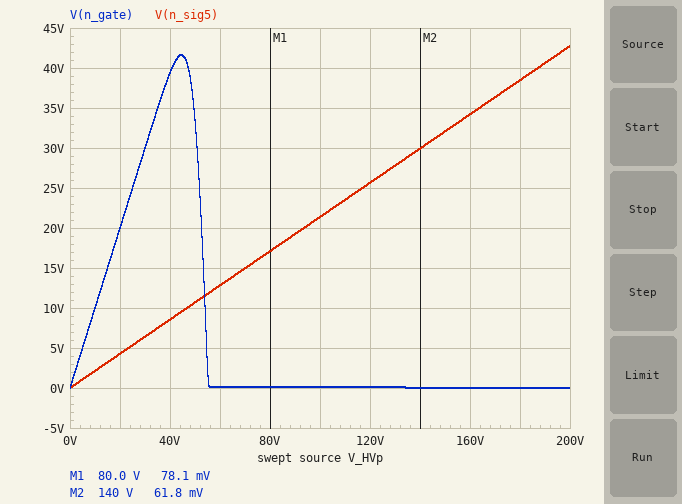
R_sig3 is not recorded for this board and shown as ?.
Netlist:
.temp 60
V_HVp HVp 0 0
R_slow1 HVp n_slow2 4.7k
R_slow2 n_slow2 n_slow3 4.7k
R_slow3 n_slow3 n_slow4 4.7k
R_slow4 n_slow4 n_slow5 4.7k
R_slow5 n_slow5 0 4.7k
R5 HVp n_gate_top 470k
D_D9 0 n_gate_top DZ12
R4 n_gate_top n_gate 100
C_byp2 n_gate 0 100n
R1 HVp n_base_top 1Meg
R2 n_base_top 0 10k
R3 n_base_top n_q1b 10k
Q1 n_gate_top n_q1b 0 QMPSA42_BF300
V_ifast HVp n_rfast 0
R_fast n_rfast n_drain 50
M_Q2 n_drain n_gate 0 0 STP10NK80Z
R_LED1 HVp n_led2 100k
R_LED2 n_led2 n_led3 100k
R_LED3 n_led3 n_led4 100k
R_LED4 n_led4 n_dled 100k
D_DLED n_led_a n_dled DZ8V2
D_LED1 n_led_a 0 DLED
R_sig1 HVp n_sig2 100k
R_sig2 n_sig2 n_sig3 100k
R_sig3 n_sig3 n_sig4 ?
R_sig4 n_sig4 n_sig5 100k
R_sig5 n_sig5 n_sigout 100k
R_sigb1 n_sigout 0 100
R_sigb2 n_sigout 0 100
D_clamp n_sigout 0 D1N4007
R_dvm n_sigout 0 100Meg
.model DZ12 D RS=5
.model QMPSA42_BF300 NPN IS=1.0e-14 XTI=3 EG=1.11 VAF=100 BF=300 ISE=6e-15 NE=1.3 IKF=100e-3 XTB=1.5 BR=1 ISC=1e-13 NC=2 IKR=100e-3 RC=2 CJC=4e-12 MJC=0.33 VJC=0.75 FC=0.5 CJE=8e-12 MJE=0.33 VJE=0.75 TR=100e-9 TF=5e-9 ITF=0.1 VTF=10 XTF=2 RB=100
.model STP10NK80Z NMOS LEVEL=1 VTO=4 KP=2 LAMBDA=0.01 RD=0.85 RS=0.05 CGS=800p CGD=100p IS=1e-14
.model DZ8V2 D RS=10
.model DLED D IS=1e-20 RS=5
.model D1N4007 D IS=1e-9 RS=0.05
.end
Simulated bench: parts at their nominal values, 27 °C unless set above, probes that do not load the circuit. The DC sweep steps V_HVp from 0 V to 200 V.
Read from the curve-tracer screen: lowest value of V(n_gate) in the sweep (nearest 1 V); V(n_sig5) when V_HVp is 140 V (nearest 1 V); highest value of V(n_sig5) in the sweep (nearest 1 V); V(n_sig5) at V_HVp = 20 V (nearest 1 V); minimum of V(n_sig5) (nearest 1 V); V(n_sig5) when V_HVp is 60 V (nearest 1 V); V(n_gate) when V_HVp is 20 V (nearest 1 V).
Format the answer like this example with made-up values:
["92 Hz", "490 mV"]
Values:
["0 V", "30 V", "43 V", "4 V", "0 V", "13 V", "20 V"]
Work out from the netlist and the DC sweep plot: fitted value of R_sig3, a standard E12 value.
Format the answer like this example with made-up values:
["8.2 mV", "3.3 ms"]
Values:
["68 kΩ"]
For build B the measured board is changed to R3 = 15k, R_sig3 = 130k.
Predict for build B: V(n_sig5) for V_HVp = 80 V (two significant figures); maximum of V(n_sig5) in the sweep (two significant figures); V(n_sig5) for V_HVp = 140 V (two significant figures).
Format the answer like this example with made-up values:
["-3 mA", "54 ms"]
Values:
["15 V", "38 V", "26 V"]
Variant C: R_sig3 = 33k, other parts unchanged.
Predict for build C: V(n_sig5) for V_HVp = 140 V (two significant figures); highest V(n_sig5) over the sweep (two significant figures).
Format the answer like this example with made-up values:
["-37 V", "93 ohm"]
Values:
["32 V", "46 V"]
